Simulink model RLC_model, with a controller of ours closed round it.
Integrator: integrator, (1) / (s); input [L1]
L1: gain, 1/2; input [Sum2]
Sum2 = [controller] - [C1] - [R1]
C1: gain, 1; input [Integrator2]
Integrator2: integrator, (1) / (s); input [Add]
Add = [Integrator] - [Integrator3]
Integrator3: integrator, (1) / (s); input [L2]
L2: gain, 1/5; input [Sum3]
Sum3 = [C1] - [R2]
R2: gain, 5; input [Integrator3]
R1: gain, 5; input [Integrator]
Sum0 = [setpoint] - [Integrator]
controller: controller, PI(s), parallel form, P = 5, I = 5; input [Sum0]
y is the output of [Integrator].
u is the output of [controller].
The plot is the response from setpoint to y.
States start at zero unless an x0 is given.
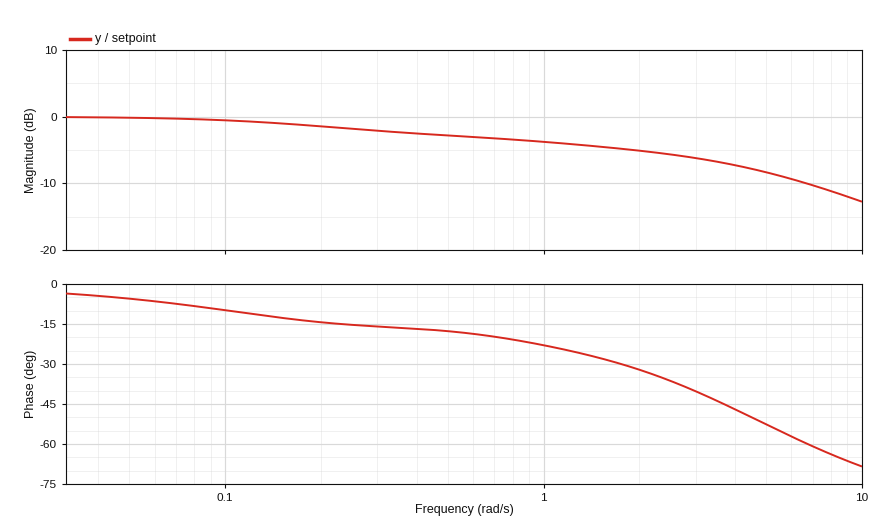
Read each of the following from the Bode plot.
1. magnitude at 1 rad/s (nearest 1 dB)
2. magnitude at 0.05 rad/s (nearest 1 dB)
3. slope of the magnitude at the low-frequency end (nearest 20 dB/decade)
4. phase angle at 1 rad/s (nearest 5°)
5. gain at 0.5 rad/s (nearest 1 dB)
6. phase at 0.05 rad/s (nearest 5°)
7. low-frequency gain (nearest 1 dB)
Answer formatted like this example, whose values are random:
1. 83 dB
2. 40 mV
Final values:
1. -4 dB
2. 0 dB
3. 0 dB/decade
4. -25°
5. -3 dB
6. -5°
7. 0 dB
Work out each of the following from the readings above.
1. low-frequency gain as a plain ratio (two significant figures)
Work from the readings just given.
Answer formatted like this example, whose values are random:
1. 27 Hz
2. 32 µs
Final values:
1. 1.0
